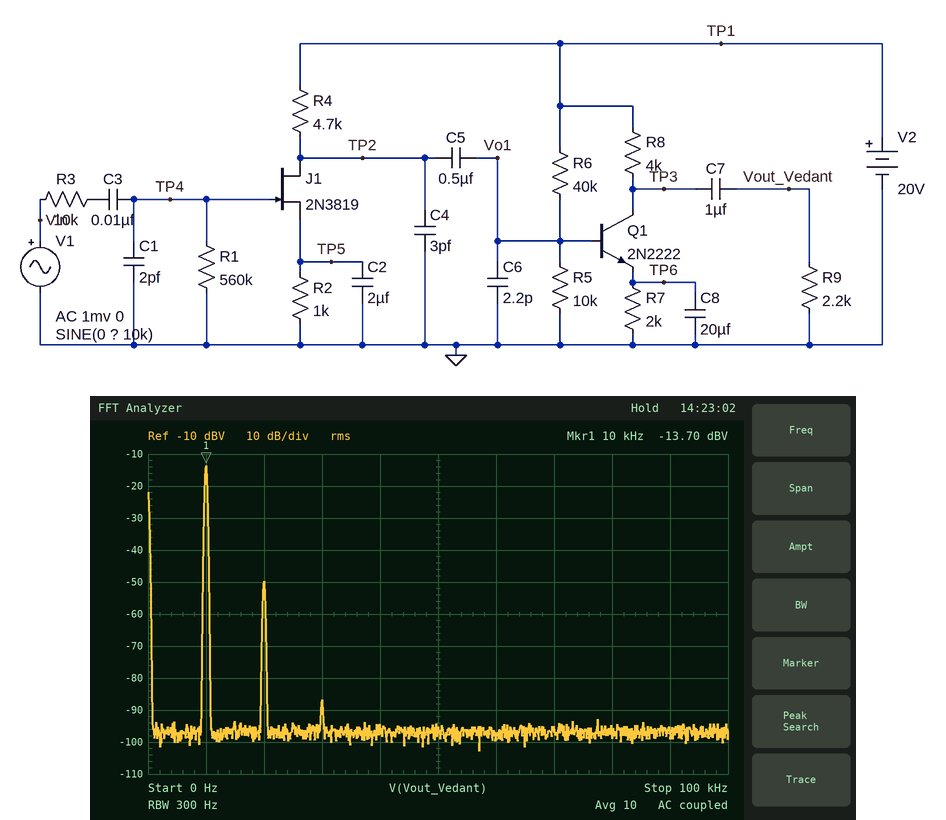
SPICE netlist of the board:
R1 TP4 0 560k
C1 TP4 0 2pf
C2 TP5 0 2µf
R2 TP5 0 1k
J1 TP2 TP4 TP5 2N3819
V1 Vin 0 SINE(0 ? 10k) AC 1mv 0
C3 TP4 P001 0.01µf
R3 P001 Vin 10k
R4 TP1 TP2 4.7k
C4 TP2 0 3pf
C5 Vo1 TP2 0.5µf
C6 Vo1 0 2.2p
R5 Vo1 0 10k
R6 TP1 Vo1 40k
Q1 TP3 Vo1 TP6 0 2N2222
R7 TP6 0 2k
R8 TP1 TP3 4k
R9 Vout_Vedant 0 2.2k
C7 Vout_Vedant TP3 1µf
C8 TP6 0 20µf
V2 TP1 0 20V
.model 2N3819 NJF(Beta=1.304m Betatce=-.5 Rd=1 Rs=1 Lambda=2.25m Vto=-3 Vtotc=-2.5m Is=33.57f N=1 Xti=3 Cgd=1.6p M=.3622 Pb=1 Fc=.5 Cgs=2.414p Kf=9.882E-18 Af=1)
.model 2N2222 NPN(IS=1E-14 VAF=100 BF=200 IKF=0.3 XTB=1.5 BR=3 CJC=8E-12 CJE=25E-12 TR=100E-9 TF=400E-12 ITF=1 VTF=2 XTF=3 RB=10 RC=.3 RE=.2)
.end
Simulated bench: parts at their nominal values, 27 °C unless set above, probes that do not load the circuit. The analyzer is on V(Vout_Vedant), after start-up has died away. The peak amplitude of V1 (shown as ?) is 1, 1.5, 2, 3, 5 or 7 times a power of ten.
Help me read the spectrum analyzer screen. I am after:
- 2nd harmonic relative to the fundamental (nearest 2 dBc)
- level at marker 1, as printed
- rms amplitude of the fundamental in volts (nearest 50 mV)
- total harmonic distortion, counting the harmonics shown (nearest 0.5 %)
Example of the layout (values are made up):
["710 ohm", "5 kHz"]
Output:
["-36 dBc", "-13.70 dBV", "200 mV", "1.5 %"]
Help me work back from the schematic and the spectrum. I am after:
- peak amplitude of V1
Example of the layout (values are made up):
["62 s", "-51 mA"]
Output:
["700 µV"]
